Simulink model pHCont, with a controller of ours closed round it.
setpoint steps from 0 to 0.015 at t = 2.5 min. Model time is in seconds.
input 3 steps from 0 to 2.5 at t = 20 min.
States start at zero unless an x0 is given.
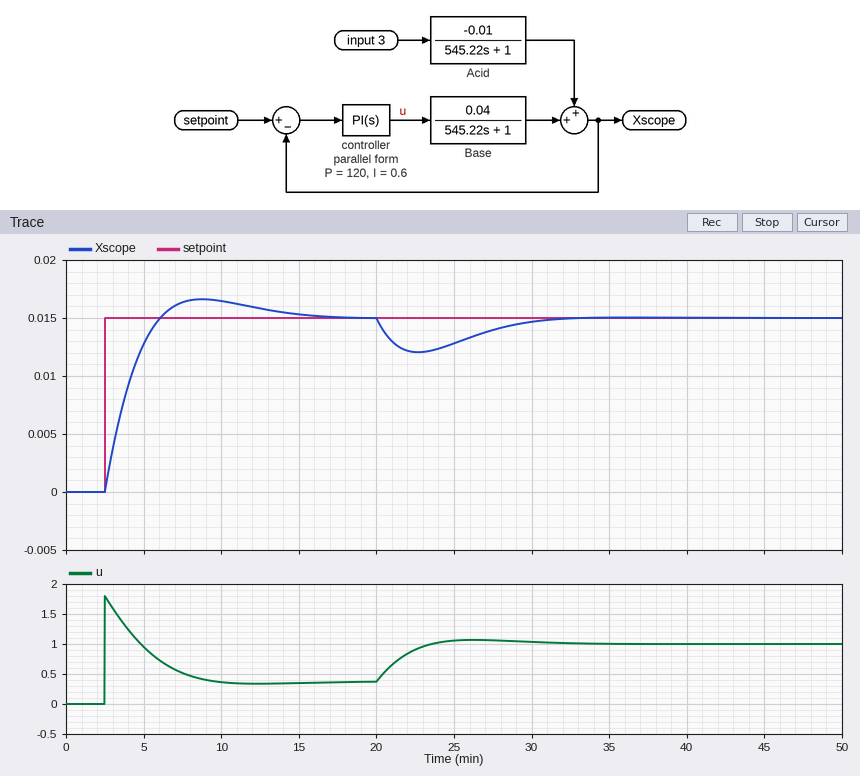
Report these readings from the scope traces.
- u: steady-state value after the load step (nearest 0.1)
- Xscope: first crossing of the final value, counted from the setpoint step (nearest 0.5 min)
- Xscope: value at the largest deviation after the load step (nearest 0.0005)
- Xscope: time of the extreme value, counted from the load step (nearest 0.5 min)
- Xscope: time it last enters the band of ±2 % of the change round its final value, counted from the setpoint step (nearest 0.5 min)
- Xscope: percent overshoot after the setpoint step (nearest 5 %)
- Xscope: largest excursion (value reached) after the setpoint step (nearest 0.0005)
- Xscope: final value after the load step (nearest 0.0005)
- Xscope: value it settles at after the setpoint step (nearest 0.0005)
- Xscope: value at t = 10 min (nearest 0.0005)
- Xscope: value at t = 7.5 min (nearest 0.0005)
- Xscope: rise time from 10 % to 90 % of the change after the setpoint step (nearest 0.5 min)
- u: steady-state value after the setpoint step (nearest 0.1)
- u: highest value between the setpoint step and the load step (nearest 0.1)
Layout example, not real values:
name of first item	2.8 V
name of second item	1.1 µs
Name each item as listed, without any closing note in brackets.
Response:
u: steady-state value after the load step	1.0
Xscope: first crossing of the final value, counted from the setpoint step	3.5 min
Xscope: value at the largest deviation after the load step	0.0120
Xscope: time of the extreme value, counted from the load step	2.5 min
Xscope: time it last enters the band of ±2 % of the change round its final value, counted from the setpoint step	12.5 min
Xscope: percent overshoot after the setpoint step	10 %
Xscope: largest excursion (value reached) after the setpoint step	0.0165
Xscope: final value after the load step	0.0150
Xscope: value it settles at after the setpoint step	0.0150
Xscope: value at t = 10 min	0.0165
Xscope: value at t = 7.5 min	0.0165
Xscope: rise time from 10 % to 90 % of the change after the setpoint step	2.5 min
u: steady-state value after the setpoint step	0.4
u: highest value between the setpoint step and the load step	1.8
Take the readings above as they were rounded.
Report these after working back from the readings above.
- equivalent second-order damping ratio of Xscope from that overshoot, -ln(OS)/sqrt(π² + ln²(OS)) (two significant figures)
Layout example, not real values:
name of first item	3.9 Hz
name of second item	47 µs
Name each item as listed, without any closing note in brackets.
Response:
equivalent second-order damping ratio of Xscope from that overshoot, -ln(OS)/sqrt(π² + ln²(OS))	0.59
